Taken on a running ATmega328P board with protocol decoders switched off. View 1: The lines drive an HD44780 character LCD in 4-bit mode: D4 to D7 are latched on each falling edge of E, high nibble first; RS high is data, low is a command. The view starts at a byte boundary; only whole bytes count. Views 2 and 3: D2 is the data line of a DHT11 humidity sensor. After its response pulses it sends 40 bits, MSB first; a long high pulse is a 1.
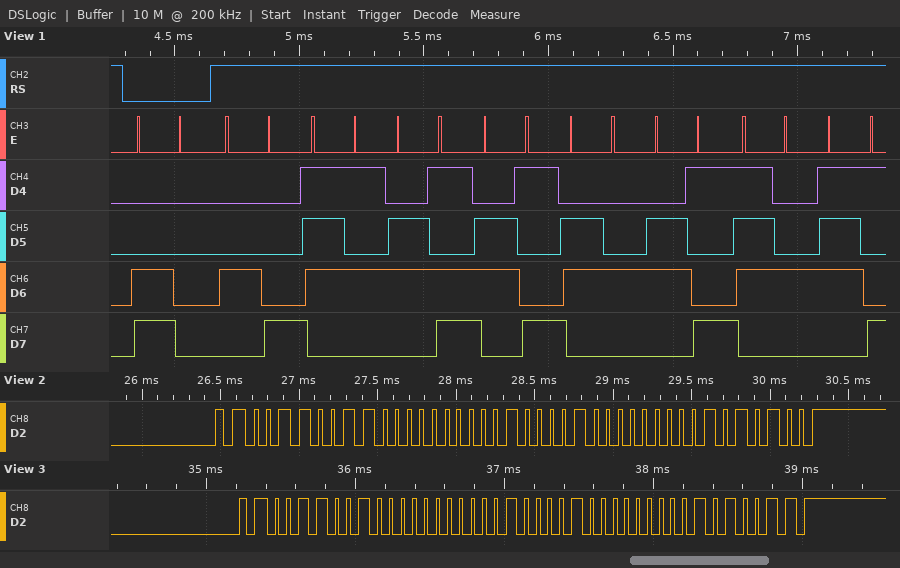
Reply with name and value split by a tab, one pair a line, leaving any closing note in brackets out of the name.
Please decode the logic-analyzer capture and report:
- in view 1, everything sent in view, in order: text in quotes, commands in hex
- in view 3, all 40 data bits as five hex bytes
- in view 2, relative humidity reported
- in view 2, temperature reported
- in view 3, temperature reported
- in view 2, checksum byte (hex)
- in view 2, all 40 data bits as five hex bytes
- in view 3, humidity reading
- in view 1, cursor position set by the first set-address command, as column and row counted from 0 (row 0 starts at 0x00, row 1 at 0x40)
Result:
in view 1, everything sent in view, in order: text in quotes, commands in hex	0xC0 "Humidity"
in view 3, all 40 data bits as five hex bytes	32 00 21 00 53
in view 2, relative humidity reported	51 %
in view 2, temperature reported	33.0 °C
in view 3, temperature reported	33.0 °C
in view 2, checksum byte	0x54
in view 2, all 40 data bits as five hex bytes	33 00 21 00 54
in view 3, humidity reading	50 %
in view 1, cursor position set by the first set-address command, as column and row counted from 0	column 0, row 1
